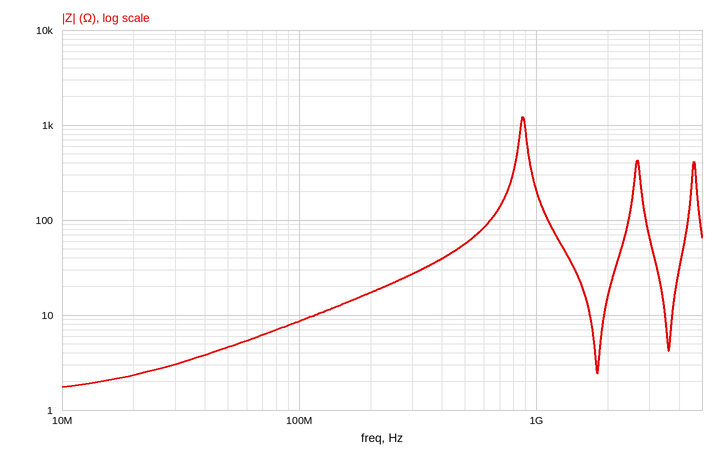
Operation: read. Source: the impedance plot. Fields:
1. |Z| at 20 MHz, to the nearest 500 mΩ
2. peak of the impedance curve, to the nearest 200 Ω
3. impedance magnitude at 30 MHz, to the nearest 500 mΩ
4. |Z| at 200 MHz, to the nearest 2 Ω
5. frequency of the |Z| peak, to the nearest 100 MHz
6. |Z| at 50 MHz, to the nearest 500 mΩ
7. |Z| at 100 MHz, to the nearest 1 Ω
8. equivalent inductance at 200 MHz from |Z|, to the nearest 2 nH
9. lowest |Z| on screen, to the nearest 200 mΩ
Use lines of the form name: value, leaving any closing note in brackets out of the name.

|Z| at 20 MHz, to the nearest 500 mΩ: 2.5 Ω
peak of the impedance curve, to the nearest 200 Ω: 1.2 kΩ
impedance magnitude at 30 MHz, to the nearest 500 mΩ: 3.0 Ω
|Z| at 200 MHz, to the nearest 2 Ω: 18 Ω
frequency of the |Z| peak, to the nearest 100 MHz: 900 MHz
|Z| at 50 MHz, to the nearest 500 mΩ: 4.5 Ω
|Z| at 100 MHz, to the nearest 1 Ω: 9 Ω
equivalent inductance at 200 MHz from |Z|, to the nearest 2 nH: 14 nH
lowest |Z| on screen, to the nearest 200 mΩ: 1.8 Ω
